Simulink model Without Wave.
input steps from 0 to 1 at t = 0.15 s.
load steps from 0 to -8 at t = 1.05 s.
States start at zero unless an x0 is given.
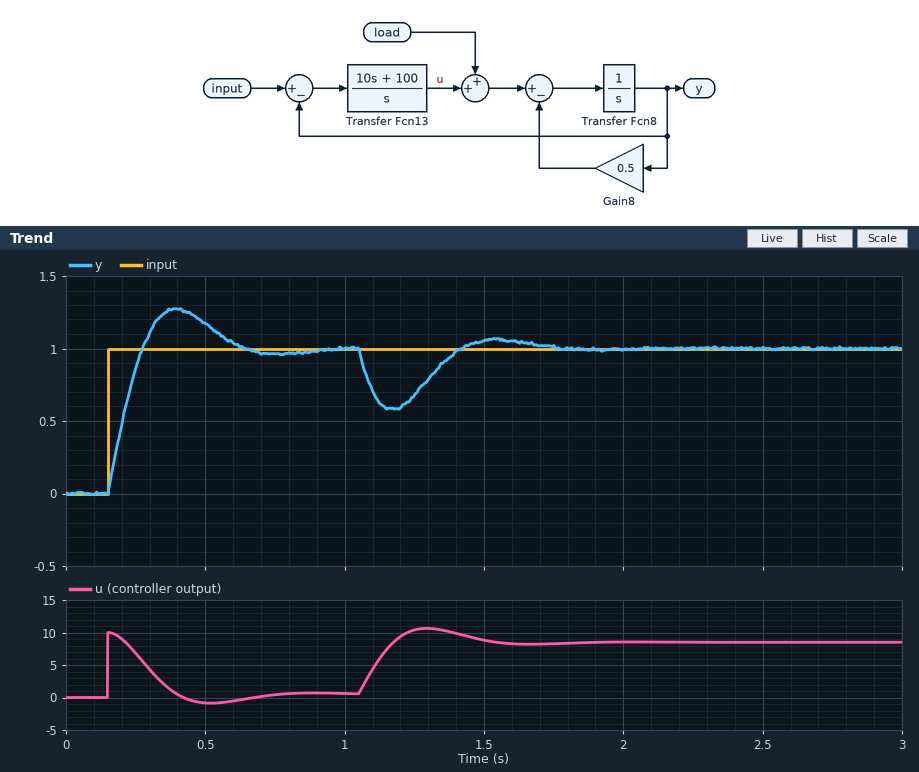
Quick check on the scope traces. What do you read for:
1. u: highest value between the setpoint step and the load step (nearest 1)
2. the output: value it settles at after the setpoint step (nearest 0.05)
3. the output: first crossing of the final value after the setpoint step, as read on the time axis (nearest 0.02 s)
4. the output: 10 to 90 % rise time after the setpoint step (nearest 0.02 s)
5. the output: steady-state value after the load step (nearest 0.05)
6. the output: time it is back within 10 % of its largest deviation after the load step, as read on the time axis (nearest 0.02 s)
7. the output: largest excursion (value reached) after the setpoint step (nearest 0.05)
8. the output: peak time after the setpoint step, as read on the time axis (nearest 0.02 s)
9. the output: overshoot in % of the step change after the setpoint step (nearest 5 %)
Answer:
10
1.00
0.28 s
0.10 s
1.00
1.64 s
1.25
0.40 s
25 %
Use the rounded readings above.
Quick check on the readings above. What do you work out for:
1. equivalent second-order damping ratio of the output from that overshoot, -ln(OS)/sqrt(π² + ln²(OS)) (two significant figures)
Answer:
0.40
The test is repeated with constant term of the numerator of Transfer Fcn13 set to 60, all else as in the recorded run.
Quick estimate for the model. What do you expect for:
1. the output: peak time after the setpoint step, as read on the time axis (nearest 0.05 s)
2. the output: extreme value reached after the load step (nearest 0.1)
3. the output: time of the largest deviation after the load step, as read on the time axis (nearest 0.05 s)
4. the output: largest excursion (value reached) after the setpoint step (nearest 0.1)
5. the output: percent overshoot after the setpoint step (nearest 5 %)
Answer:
0.45 s
0.5
1.20 s
1.2
20 %
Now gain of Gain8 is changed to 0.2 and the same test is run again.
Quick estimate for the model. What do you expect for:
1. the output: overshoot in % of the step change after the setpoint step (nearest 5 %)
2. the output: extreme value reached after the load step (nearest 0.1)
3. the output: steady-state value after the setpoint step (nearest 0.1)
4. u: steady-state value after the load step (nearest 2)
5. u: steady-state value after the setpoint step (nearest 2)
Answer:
30 %
0.6
1.0
8
0
